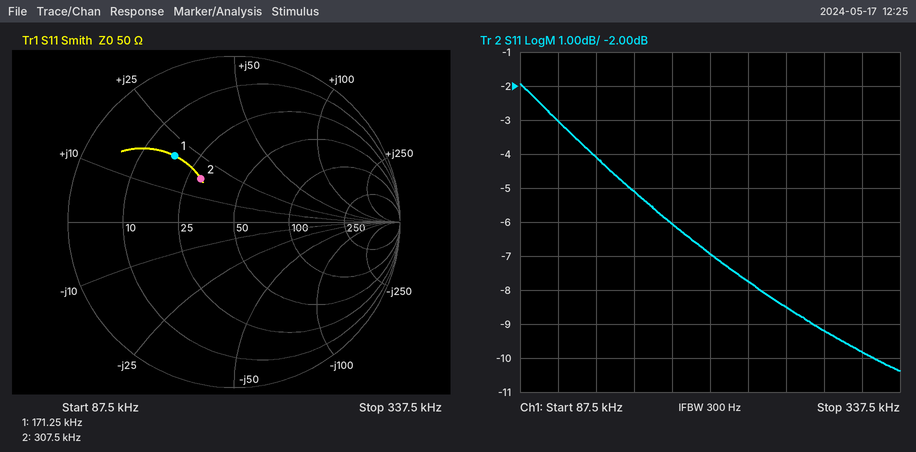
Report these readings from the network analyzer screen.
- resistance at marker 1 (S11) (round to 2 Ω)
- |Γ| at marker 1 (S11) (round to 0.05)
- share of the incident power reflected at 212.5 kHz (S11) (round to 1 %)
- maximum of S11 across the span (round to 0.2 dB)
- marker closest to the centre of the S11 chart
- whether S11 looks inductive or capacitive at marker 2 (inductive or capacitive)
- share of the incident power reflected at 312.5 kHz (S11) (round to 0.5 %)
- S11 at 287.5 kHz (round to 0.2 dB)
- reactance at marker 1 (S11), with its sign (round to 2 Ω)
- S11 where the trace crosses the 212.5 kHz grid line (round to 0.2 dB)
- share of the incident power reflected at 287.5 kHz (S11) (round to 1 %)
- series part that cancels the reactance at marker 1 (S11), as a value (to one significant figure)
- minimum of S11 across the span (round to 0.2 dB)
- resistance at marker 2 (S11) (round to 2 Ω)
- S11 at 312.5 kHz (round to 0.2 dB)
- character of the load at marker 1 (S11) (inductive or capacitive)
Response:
18 Ω
0.55
20 %
-2.0 dB
marker 2
inductive
10.5 %
-9.2 dB
+20 Ω
-7.0 dB
12 %
50 nF
-10.4 dB
30 Ω
-9.8 dB
inductive
